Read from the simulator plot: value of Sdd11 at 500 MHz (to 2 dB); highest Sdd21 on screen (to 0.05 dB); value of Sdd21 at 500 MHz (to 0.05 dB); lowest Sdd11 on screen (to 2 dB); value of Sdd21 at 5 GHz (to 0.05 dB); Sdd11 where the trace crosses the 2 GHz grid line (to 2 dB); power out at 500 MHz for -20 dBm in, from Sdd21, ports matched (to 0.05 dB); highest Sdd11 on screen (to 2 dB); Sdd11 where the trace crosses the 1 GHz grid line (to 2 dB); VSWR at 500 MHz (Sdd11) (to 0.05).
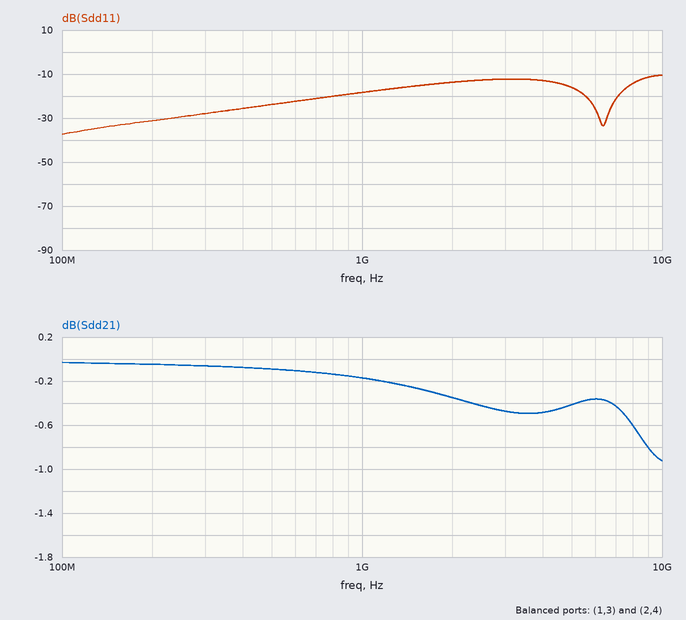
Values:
-24 dB
-0.05 dB
-0.10 dB
-38 dB
-0.40 dB
-14 dB
-20.10 dBm
-10 dB
-18 dB
1.15
